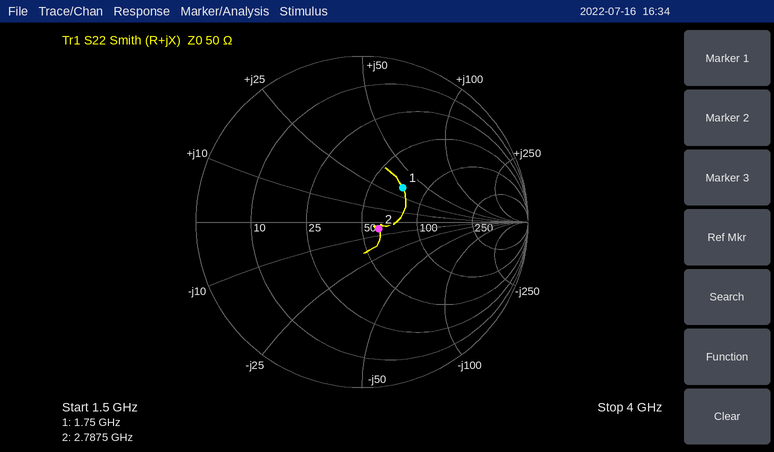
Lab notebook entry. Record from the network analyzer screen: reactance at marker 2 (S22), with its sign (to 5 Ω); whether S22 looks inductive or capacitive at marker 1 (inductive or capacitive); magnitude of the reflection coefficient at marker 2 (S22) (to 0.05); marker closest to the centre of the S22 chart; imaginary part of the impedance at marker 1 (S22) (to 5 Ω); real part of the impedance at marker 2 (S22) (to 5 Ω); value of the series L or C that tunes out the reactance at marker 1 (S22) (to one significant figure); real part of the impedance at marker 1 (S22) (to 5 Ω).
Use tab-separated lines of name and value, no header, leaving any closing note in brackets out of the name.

reactance at marker 2 (S22), with its sign	-5 Ω
whether S22 looks inductive or capacitive at marker 1	inductive
magnitude of the reflection coefficient at marker 2 (S22)	0.10
marker closest to the centre of the S22 chart	marker 2
imaginary part of the impedance at marker 1 (S22)	+35 Ω
real part of the impedance at marker 2 (S22)	60 Ω
value of the series L or C that tunes out the reactance at marker 1 (S22)	3 pF
real part of the impedance at marker 1 (S22)	75 Ω
